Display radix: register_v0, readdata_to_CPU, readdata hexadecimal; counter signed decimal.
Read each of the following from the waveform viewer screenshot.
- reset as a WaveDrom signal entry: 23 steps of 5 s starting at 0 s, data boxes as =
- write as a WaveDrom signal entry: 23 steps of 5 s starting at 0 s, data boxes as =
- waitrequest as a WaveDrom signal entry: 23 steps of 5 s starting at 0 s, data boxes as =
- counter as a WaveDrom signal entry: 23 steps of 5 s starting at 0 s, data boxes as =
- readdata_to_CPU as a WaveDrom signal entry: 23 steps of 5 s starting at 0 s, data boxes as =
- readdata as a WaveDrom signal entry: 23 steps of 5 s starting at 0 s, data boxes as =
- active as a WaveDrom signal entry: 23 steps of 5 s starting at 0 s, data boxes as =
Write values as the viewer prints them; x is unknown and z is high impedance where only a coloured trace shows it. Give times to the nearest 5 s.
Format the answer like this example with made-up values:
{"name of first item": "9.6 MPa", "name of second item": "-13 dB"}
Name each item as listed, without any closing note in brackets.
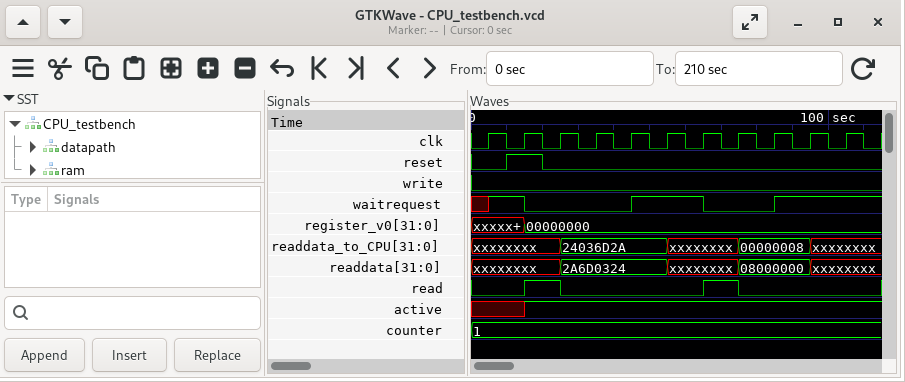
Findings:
{"reset as a WaveDrom signal entry: 23 steps of 5 s starting at 0 s, data boxes as =": "{name: 'reset', wave: '0.1.0..................'}", "write as a WaveDrom signal entry: 23 steps of 5 s starting at 0 s, data boxes as =": "{name: 'write', wave: '0......................'}", "waitrequest as a WaveDrom signal entry: 23 steps of 5 s starting at 0 s, data boxes as =": "{name: 'waitrequest', wave: 'x1.0.....1...0...1.....'}", "counter as a WaveDrom signal entry: 23 steps of 5 s starting at 0 s, data boxes as =": "{name: 'counter', wave: '=......................', data: '1'}", "readdata_to_CPU as a WaveDrom signal entry: 23 steps of 5 s starting at 0 s, data boxes as =": "{name: 'readdata_to_CPU', wave: 'x....=.....x...=...x...', data: '24036D2A 00000008'}", "readdata as a WaveDrom signal entry: 23 steps of 5 s starting at 0 s, data boxes as =": "{name: 'readdata', wave: 'x....=.....x...=...x...', data: '2A6D0324 08000000'}", "active as a WaveDrom signal entry: 23 steps of 5 s starting at 0 s, data boxes as =": "{name: 'active', wave: 'x..1...................'}"}
